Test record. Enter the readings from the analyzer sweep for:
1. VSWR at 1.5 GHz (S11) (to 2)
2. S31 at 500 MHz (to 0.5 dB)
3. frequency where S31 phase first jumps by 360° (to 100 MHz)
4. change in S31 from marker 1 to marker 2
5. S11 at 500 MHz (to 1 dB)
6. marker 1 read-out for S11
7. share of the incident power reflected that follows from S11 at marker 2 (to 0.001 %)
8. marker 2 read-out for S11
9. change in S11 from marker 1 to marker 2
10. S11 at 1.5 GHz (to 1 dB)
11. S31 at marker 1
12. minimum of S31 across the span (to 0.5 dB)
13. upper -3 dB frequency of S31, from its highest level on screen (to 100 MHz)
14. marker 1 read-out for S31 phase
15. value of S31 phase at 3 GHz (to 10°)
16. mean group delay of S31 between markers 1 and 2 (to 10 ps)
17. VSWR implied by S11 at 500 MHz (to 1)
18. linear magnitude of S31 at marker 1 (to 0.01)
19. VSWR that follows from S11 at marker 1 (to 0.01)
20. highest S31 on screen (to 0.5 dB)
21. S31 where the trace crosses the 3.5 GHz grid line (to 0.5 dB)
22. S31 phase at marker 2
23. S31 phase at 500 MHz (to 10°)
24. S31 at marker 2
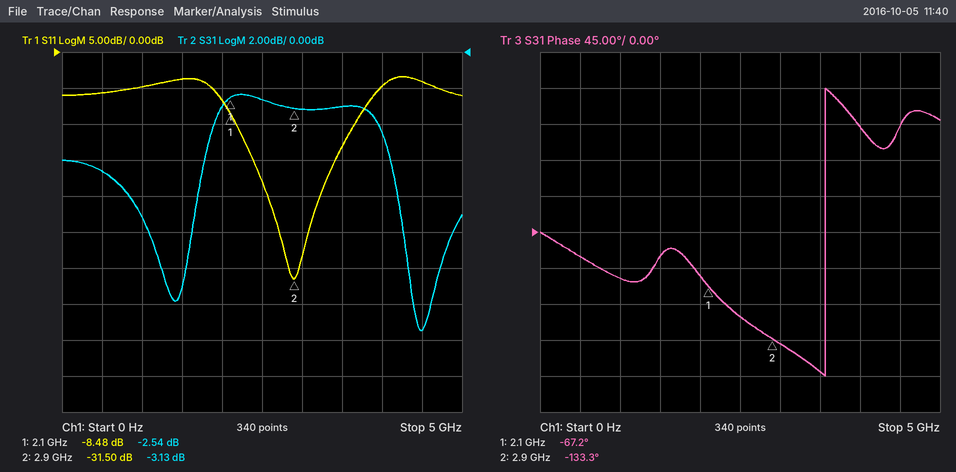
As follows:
4
-6.5 dB
3.6 GHz
-0.59 dB
-6 dB
-8.48 dB
0.071 %
-31.50 dB
-23.02 dB
-4 dB
-2.54 dB
-15.5 dB
4.1 GHz
-67.2°
-140°
230 ps
3
0.75
2.21
-2.5 dB
-3.0 dB
-133.3°
-30°
-3.13 dB
